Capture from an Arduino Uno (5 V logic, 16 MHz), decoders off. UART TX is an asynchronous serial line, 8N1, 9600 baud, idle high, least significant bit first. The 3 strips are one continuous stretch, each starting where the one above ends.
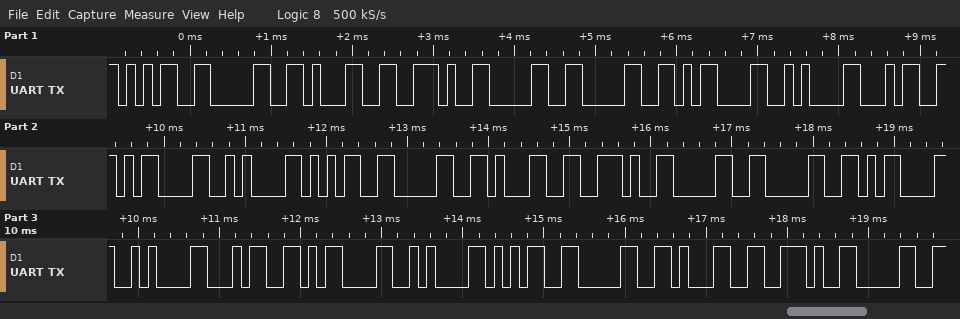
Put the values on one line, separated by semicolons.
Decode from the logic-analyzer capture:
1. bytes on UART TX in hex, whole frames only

35 30 31 2E 30 30 0D 0A 34 0D 0A 35 30 31 2E 30 30 0D 0A 34 0D 0A 35 30 31 2E 30
